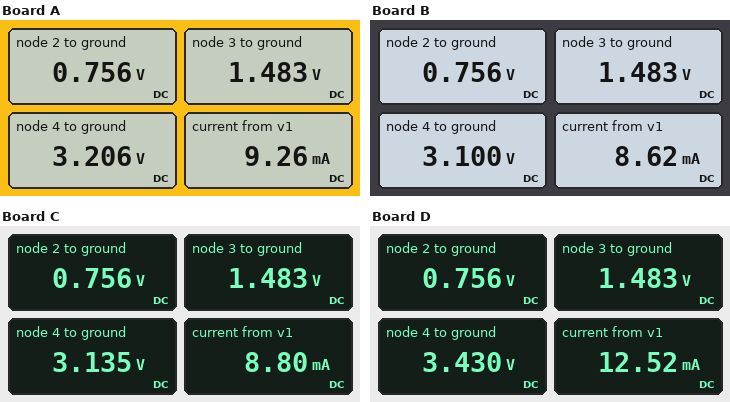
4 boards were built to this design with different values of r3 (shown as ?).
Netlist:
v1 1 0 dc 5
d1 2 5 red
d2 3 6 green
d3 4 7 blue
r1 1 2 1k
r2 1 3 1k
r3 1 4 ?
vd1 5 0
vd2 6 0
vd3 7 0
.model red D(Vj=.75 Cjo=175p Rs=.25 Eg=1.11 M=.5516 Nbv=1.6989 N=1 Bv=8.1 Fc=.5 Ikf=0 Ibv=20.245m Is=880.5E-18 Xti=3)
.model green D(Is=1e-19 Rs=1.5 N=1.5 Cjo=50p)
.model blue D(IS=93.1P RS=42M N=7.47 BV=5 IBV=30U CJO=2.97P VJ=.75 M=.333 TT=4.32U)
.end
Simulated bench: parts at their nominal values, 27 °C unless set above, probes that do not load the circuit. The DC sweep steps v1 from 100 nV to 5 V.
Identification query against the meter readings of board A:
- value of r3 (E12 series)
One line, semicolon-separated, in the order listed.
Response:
1.2 kΩ
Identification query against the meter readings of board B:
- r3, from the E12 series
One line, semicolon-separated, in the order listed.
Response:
2.2 kΩ
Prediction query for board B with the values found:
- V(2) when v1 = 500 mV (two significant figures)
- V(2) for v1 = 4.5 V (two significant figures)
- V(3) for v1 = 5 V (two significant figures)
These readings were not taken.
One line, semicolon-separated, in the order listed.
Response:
500 mV; 750 mV; 1.5 V
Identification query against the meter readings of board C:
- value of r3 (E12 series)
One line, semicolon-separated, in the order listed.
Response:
1.8 kΩ
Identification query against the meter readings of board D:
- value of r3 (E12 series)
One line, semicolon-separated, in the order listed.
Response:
330 Ω
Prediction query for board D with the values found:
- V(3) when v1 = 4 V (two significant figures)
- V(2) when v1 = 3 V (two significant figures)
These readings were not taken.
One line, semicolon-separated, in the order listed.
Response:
1.5 V; 740 mV
